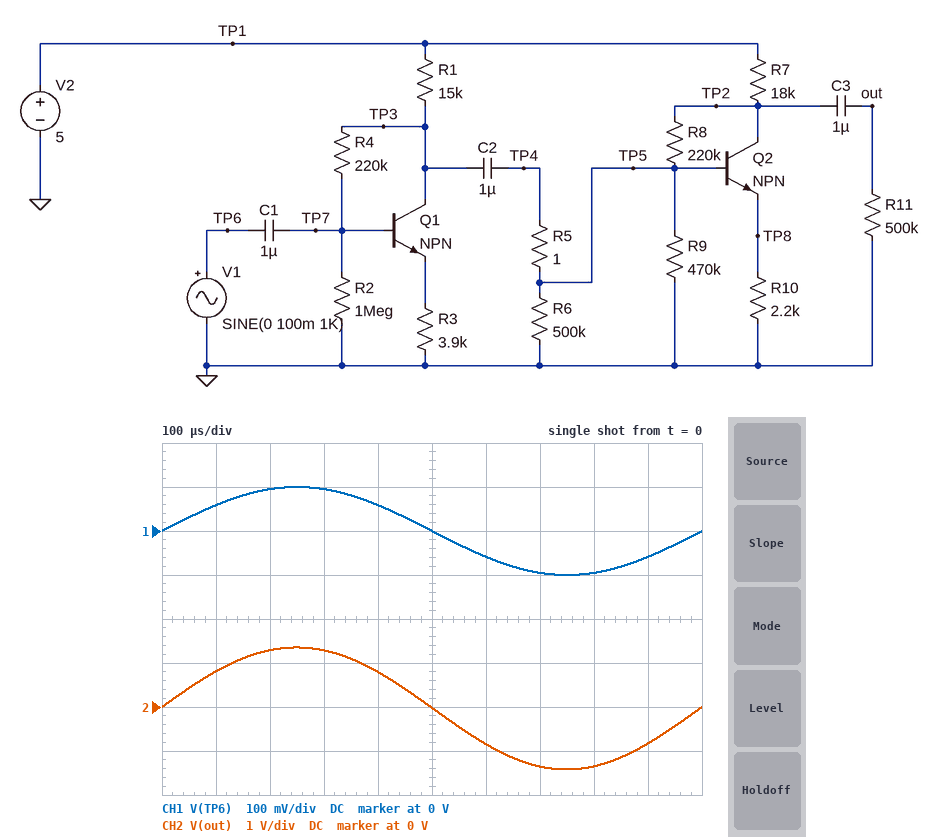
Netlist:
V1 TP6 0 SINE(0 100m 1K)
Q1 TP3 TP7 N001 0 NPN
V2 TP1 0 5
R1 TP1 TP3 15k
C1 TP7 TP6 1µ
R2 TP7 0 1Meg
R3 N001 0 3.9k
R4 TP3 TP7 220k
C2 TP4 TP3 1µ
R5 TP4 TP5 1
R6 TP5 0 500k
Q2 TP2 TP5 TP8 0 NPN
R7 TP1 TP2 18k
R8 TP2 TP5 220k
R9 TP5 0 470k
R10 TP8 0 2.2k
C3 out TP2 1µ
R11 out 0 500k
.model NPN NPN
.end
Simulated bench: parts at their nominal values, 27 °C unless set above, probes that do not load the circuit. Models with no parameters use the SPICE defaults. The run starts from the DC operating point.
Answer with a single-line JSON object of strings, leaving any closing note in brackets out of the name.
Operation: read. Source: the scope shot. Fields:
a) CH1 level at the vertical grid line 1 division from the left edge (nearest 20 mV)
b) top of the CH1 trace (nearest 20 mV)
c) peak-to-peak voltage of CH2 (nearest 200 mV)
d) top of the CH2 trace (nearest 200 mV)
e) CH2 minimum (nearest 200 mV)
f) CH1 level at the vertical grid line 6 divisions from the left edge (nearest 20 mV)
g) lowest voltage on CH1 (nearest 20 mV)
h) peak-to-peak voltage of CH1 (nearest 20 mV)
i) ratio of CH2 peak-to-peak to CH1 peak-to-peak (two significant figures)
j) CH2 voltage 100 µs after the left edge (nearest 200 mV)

{"CH1 level at the vertical grid line 1 division from the left edge": "60 mV", "top of the CH1 trace": "100 mV", "peak-to-peak voltage of CH2": "2.8 V", "top of the CH2 trace": "1.4 V", "CH2 minimum": "-1.4 V", "CH1 level at the vertical grid line 6 divisions from the left edge": "-60 mV", "lowest voltage on CH1": "-100 mV", "peak-to-peak voltage of CH1": "200 mV", "ratio of CH2 peak-to-peak to CH1 peak-to-peak": "14", "CH2 voltage 100 µs after the left edge": "800 mV"}
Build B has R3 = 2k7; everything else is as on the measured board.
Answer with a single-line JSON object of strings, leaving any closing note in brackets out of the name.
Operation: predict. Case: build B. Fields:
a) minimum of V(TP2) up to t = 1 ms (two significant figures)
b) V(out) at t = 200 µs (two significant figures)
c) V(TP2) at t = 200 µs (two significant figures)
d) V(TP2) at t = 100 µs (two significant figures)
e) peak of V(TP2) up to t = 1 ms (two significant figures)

{"minimum of V(TP2) up to t = 1 ms": "660 mV", "V(out) at t = 200 µs": "1.8 V", "V(TP2) at t = 200 µs": "4.1 V", "V(TP2) at t = 100 µs": "3.5 V", "peak of V(TP2) up to t = 1 ms": "4.2 V"}
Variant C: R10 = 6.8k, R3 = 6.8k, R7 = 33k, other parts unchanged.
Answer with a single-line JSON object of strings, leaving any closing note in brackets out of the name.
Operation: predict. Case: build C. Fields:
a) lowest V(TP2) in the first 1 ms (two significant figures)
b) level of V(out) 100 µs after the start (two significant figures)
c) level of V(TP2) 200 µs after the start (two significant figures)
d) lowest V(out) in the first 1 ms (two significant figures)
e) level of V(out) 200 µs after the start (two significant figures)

{"lowest V(TP2) in the first 1 ms": "1.9 V", "level of V(out) 100 µs after the start": "300 mV", "level of V(TP2) 200 µs after the start": "2.9 V", "lowest V(out) in the first 1 ms": "-520 mV", "level of V(out) 200 µs after the start": "480 mV"}
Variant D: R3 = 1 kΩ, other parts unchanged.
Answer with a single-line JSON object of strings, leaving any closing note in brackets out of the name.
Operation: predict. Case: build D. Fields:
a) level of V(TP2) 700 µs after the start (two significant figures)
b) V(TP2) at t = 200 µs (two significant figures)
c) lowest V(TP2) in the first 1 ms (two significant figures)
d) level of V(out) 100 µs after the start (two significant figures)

{"level of V(TP2) 700 µs after the start": "700 mV", "V(TP2) at t = 200 µs": "4.6 V", "lowest V(TP2) in the first 1 ms": "660 mV", "level of V(out) 100 µs after the start": "2.3 V"}
